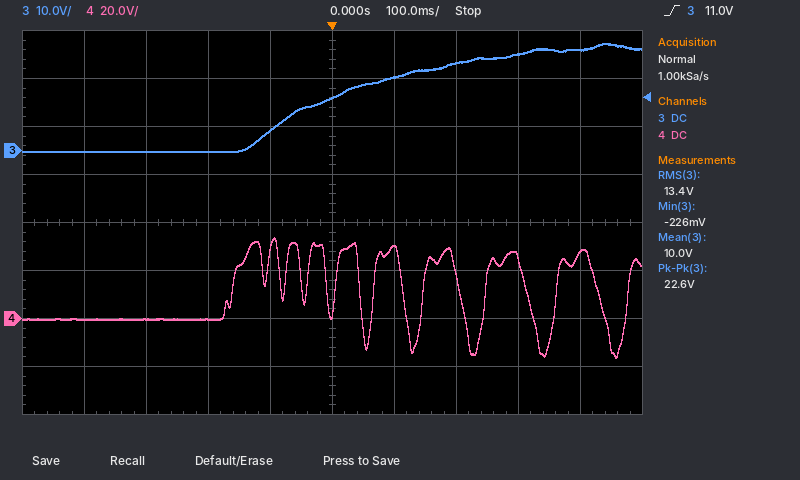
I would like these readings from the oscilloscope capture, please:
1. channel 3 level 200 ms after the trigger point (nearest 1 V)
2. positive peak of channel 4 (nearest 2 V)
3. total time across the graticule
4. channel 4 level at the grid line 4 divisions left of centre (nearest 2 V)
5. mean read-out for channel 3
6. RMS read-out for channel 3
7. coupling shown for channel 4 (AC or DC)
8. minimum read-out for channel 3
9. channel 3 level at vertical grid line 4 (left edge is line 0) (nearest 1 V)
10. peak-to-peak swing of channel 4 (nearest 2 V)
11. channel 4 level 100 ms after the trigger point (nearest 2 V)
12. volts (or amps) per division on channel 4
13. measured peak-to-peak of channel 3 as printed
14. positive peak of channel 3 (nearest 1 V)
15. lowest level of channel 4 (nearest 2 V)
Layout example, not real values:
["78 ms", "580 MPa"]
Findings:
["18 V", "34 V", "1 s", "0 V", "10.0 V", "13.4 V", "DC", "-226 mV", "4 V", "50 V", "30 V", "20 V", "22.6 V", "22 V", "-16 V"]
